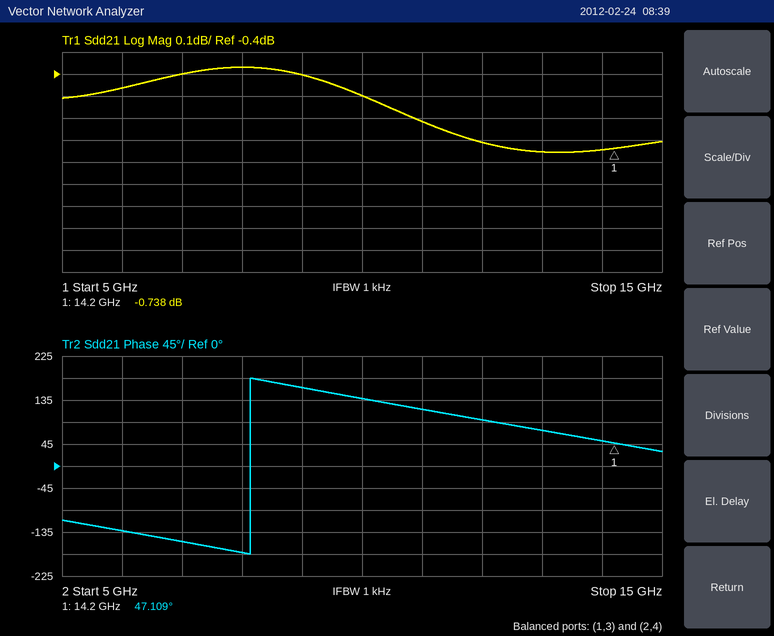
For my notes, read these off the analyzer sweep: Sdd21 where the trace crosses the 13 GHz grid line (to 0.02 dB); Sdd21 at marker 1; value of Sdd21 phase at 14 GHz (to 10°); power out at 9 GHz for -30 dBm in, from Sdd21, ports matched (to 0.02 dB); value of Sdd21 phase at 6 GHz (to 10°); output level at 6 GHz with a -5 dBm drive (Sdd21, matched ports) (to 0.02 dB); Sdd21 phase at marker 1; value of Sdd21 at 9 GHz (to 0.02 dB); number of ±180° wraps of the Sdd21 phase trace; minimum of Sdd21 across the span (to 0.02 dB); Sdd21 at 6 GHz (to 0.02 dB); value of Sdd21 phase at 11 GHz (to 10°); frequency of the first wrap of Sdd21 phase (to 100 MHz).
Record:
-0.76 dB
-0.738 dB
50°
-30.40 dBm
-130°
-5.46 dBm
47.109°
-0.40 dB
1
-0.76 dB
-0.46 dB
120°
8.1 GHz
